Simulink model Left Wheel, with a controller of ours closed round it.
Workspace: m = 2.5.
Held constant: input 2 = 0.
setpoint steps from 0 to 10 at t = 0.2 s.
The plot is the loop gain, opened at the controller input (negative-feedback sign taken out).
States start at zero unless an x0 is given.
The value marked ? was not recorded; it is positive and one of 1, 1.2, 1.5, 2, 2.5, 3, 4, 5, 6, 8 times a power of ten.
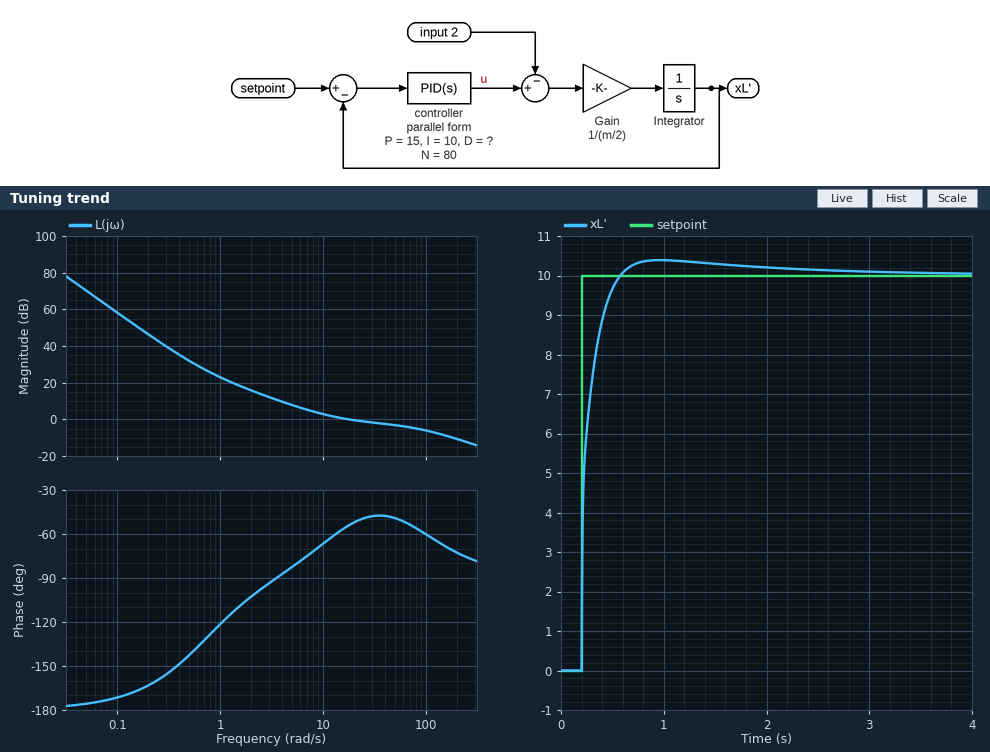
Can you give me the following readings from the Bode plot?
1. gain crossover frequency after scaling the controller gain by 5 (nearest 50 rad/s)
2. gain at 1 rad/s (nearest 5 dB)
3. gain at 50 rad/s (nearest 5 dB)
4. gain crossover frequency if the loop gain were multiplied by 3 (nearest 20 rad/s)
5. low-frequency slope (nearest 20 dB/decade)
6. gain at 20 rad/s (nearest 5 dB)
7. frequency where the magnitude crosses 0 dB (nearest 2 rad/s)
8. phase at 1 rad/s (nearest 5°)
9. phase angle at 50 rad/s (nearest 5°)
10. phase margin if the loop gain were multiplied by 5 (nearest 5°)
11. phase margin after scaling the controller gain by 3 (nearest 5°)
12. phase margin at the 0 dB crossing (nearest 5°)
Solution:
300 rad/s
25 dB
-5 dB
180 rad/s
-40 dB/decade
0 dB
18 rad/s
-120°
-50°
100°
110°
125°
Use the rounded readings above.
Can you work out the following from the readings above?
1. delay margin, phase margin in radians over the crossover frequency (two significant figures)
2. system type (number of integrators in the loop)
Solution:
0.12 s
2
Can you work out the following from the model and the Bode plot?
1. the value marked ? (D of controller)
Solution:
0.8
